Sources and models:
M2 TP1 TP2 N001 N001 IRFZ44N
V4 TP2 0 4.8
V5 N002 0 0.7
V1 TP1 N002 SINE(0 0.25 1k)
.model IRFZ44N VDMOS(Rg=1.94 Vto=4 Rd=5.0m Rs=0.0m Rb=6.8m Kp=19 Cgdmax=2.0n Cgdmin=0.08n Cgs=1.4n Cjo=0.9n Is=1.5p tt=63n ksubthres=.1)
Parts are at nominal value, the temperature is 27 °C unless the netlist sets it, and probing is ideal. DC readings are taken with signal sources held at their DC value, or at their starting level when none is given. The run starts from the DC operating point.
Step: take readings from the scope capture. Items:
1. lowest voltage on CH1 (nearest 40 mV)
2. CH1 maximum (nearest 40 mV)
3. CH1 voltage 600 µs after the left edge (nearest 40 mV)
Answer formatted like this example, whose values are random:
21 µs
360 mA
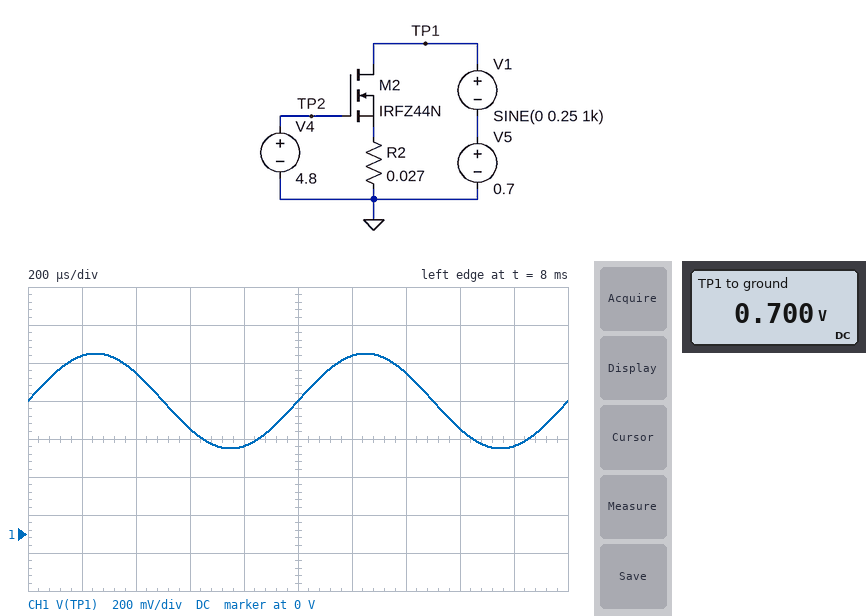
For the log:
440 mV
960 mV
560 mV
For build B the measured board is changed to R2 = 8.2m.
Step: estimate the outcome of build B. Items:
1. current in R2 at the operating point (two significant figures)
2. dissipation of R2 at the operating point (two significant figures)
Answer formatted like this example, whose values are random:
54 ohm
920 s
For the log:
5.3 A
230 mW
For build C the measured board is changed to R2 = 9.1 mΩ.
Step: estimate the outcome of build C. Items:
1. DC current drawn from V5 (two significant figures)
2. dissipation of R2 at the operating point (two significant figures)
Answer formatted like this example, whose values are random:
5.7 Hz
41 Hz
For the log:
5.2 A
250 mW
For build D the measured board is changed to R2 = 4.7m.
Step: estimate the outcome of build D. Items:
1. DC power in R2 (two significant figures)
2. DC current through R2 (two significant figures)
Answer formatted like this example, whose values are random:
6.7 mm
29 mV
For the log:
140 mW
5.5 A
